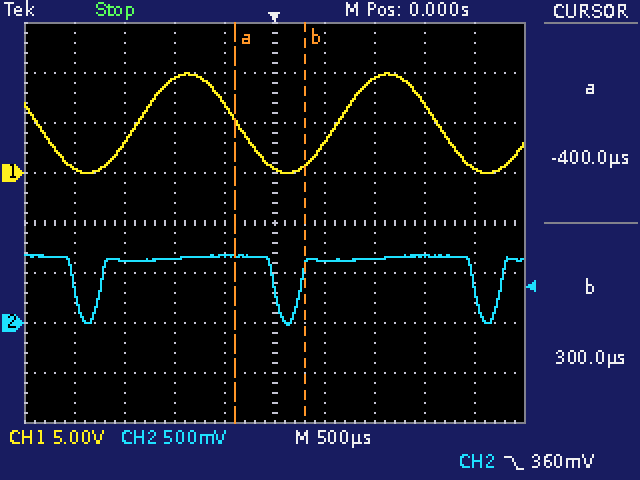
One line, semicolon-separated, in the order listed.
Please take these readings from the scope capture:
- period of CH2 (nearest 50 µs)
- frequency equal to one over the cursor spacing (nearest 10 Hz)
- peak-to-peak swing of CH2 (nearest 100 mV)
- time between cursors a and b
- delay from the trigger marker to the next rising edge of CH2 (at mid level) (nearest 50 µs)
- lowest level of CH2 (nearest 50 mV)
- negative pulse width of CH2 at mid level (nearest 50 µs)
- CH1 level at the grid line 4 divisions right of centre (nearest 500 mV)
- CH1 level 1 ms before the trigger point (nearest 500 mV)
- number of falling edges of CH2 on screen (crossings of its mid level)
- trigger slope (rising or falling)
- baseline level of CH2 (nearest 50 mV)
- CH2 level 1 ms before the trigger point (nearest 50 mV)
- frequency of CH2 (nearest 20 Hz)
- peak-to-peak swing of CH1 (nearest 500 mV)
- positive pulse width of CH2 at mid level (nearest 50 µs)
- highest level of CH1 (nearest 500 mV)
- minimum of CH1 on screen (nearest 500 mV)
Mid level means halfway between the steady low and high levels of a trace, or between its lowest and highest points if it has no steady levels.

2.00 ms; 1.43 kHz; 700 mV; 700 µs; 250 µs; 0 mV; 250 µs; 500 mV; 9.5 V; 3; falling; 650 mV; 650 mV; 500 Hz; 10.0 V; 1.75 ms; 10.0 V; 0.0 V
